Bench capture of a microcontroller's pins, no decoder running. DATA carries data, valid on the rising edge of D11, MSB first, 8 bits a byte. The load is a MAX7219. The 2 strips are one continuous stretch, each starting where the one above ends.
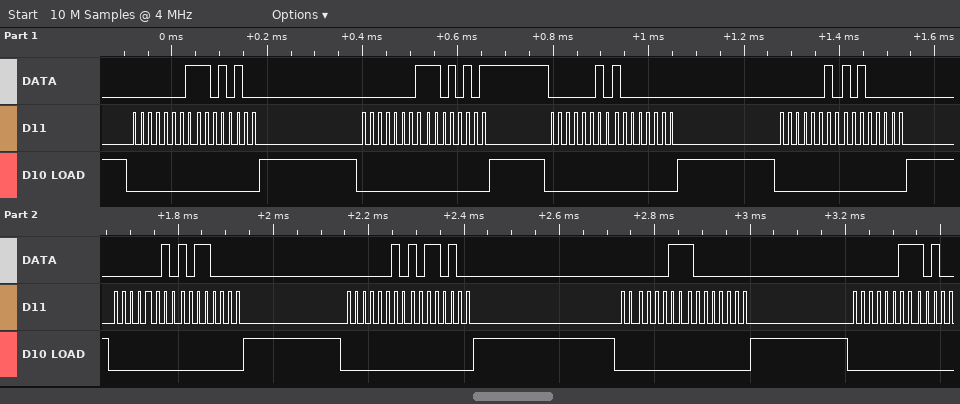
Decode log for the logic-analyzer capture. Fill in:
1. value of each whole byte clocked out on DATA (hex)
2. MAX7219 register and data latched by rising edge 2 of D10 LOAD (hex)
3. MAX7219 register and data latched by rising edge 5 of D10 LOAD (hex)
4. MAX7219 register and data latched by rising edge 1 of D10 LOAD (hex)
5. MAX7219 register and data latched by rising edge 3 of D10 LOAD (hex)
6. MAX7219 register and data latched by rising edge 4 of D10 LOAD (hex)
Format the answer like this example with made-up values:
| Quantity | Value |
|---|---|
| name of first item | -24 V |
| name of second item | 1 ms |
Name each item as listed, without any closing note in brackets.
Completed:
| Quantity | Value |
|---|---|
| value of each whole byte clocked out on DATA | 0x01 0xD4 0x01 0xD5 0x02 0x80 0x02 0xA0 0x02 0xB0 0x02 0xB4 0x03 0x80 0x03 |
| MAX7219 register and data latched by rising edge 2 of D10 LOAD | register 0x1, data 0xD5 |
| MAX7219 register and data latched by rising edge 5 of D10 LOAD | register 0x2, data 0xB0 |
| MAX7219 register and data latched by rising edge 1 of D10 LOAD | register 0x1, data 0xD4 |
| MAX7219 register and data latched by rising edge 3 of D10 LOAD | register 0x2, data 0x80 |
| MAX7219 register and data latched by rising edge 4 of D10 LOAD | register 0x2, data 0xA0 |
